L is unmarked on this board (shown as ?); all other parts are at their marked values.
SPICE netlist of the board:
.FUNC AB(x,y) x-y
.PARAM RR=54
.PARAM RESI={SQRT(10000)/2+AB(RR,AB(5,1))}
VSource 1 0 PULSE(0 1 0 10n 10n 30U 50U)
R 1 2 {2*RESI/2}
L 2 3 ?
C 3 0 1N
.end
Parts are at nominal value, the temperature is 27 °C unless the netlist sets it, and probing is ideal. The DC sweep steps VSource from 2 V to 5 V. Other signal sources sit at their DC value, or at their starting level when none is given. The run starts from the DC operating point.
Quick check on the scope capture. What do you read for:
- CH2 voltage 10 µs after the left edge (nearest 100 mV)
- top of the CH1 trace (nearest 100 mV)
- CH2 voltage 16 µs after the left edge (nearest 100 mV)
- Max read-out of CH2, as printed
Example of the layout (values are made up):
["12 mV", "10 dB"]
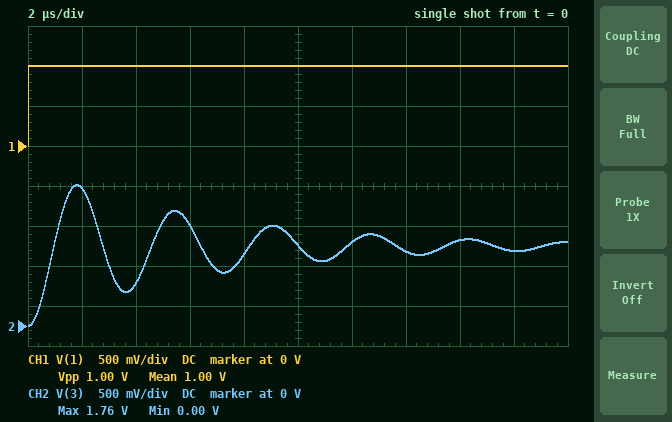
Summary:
["1.0 V", "1.0 V", "1.1 V", "1.76 V"]
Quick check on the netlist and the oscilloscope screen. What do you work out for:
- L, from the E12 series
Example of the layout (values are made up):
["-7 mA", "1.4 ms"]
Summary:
["330 µH"]
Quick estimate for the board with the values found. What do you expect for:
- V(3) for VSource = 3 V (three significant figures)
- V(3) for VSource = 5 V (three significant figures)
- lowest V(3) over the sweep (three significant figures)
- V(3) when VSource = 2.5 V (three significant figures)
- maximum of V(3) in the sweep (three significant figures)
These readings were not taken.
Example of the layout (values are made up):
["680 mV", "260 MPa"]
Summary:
["3.00 V", "5.00 V", "2.00 V", "2.50 V", "5.00 V"]
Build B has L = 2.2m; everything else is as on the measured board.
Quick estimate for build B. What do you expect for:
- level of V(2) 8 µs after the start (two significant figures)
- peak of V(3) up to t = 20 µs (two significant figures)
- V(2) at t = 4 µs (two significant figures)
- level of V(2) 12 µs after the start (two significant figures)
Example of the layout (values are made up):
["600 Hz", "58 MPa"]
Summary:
["1.0 V", "1.9 V", "970 mV", "950 mV"]
